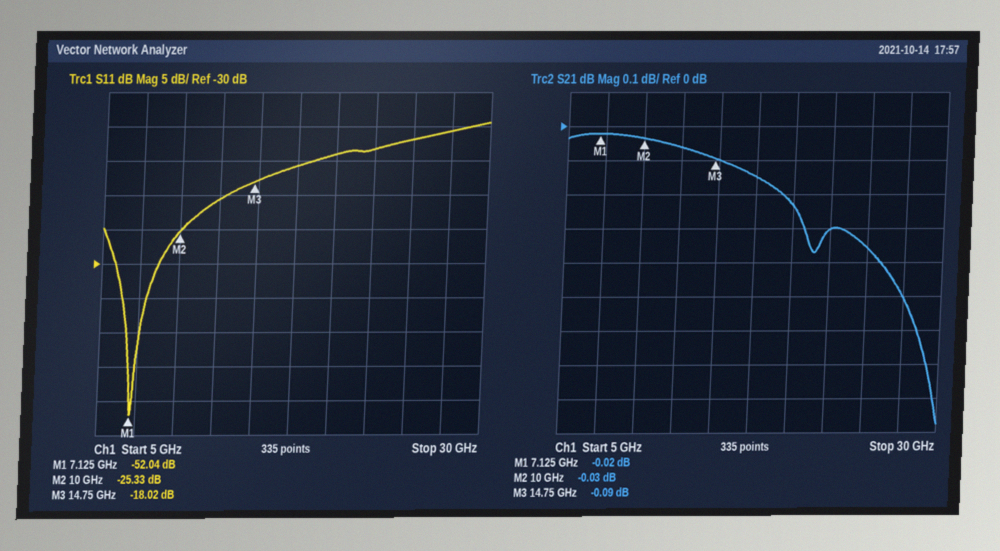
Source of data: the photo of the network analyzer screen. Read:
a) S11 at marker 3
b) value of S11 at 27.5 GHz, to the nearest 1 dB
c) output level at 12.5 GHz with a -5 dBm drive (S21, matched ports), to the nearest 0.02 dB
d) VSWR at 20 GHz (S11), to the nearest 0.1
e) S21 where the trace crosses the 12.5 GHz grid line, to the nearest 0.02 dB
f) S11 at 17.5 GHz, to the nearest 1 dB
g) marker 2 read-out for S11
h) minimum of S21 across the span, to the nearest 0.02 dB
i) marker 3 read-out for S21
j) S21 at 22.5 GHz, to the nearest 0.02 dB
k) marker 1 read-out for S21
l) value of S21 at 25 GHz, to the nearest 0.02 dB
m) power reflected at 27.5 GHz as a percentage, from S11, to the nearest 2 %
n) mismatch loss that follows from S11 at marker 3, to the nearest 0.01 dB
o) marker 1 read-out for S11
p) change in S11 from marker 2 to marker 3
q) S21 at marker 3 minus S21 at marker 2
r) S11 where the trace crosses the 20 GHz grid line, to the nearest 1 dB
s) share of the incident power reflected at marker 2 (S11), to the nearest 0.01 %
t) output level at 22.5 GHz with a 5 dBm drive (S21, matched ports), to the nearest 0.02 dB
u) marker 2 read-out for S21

-18.02 dB
-11 dB
-5.06 dBm
1.5
-0.06 dB
-16 dB
-25.33 dB
-0.88 dB
-0.09 dB
-0.30 dB
-0.02 dB
-0.36 dB
8 %
0.07 dB
-52.04 dB
7.31 dB
-0.06 dB
-14 dB
0.29 %
4.70 dBm
-0.03 dB
